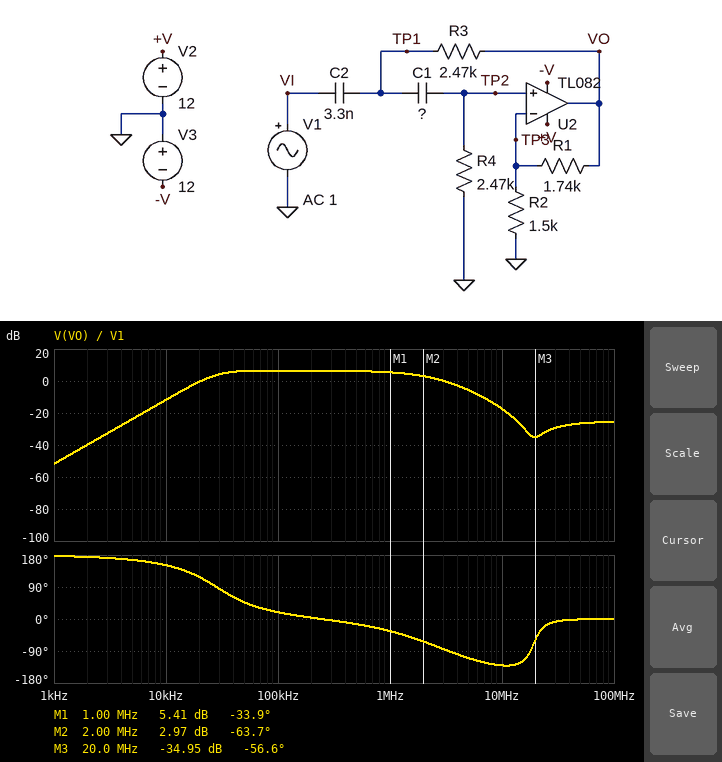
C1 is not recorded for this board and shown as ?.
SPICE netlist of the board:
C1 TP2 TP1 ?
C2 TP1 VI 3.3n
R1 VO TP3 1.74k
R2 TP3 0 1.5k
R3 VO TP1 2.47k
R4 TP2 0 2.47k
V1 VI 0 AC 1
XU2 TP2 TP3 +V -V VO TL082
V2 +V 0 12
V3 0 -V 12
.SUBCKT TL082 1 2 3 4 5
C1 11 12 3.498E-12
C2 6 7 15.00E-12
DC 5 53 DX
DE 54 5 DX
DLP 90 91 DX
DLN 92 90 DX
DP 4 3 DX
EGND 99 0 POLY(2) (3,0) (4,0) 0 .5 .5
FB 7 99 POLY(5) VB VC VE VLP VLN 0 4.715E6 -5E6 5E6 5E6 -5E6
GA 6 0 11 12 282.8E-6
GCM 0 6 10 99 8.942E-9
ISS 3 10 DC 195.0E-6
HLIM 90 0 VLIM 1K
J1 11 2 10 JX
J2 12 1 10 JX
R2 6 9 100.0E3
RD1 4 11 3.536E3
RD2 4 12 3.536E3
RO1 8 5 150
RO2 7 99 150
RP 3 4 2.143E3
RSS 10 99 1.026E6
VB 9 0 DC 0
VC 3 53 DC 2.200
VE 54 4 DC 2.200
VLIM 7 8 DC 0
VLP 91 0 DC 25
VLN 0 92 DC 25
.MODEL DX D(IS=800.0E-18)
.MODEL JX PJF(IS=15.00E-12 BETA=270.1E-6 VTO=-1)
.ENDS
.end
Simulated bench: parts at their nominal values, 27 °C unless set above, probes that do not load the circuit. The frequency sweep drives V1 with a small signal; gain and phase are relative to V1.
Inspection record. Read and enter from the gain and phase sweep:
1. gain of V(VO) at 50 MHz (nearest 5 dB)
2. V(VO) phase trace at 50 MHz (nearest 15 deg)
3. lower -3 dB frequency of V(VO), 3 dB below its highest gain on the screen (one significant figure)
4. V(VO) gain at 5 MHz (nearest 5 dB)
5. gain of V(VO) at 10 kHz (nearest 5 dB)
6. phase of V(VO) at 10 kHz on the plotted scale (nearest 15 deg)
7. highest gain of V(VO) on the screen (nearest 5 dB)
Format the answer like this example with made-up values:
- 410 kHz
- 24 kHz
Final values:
- -25 dB
- 0 deg
- 30 kHz
- -5 dB
- -10 dB
- 150 deg
- 5 dB
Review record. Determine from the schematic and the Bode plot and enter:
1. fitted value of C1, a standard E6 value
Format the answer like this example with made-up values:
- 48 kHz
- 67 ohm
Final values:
- 1.5 nF
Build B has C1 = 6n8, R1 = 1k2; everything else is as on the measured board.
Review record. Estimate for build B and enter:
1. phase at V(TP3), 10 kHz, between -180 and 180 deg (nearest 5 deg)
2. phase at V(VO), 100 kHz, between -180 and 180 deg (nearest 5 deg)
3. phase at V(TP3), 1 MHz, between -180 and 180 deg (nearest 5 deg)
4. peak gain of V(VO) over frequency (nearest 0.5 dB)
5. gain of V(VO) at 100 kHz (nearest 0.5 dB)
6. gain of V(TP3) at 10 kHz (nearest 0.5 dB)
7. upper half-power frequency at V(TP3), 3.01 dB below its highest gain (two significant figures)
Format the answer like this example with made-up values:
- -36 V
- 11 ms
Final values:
- 120 deg
- 5 deg
- -30 deg
- 6.5 dB
- 5.0 dB
- -4.0 dB
- 1.6 MHz
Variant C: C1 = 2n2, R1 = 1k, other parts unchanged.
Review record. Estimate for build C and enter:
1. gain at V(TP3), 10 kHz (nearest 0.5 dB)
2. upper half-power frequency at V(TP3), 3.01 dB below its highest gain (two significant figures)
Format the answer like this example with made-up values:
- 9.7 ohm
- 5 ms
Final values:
- -15.5 dB
- 2.4 MHz
